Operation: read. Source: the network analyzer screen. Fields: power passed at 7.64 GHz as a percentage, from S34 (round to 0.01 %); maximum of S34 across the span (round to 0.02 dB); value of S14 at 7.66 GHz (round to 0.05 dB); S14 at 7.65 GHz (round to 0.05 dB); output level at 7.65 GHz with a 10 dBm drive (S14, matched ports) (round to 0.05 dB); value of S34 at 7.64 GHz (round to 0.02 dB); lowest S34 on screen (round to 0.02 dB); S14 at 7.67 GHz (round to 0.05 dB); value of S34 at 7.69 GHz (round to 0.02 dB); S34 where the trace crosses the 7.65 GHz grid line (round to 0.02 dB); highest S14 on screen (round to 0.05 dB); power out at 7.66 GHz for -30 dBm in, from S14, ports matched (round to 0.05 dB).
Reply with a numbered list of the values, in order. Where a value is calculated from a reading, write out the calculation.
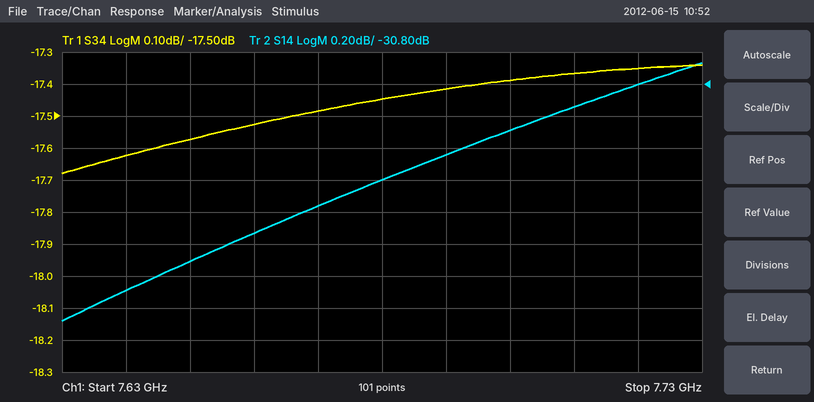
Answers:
1. 10^(-17.62/10) ≈ 1.73 %
2. -17.34 dB
3. -31.75 dB
4. -31.90 dB
5. 10 dBm + (-31.90 dB) = -21.90 dBm
6. -17.62 dB
7. -17.68 dB
8. -31.55 dB
9. -17.42 dB
10. -17.58 dB
11. -30.65 dB
12. -30 dBm + (-31.75 dB) = -61.75 dBm
